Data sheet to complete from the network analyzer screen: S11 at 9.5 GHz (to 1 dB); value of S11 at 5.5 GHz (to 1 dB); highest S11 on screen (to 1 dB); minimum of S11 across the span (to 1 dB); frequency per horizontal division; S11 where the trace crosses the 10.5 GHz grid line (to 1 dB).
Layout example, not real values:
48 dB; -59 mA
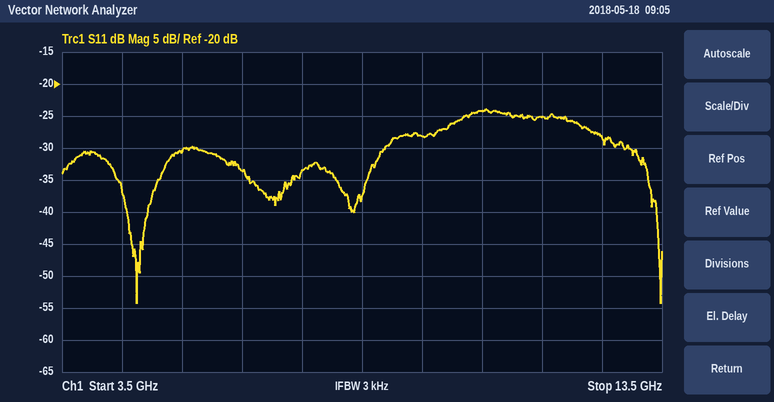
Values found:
-28 dB; -31 dB; -24 dB; -54 dB; 1 GHz; -24 dB
